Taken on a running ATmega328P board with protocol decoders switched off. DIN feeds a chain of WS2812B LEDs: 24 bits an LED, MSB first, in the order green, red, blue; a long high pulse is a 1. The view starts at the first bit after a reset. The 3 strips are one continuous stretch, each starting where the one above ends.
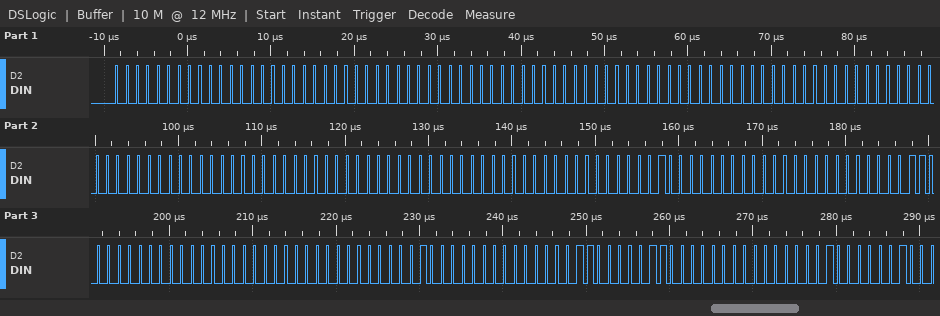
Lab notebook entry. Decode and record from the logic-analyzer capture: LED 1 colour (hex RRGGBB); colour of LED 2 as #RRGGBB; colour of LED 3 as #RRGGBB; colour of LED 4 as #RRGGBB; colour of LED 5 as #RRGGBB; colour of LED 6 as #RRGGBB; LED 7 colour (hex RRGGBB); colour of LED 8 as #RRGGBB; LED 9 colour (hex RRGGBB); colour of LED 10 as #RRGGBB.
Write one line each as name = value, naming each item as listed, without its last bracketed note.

LED 1 colour = #000000
colour of LED 2 as #RRGGBB = #000000
colour of LED 3 as #RRGGBB = #000000
colour of LED 4 as #RRGGBB = #000000
colour of LED 5 as #RRGGBB = #000000
colour of LED 6 as #RRGGBB = #040000
LED 7 colour = #060000
colour of LED 8 as #RRGGBB = #000001
LED 9 colour = #030006
colour of LED 10 as #RRGGBB = #020004
